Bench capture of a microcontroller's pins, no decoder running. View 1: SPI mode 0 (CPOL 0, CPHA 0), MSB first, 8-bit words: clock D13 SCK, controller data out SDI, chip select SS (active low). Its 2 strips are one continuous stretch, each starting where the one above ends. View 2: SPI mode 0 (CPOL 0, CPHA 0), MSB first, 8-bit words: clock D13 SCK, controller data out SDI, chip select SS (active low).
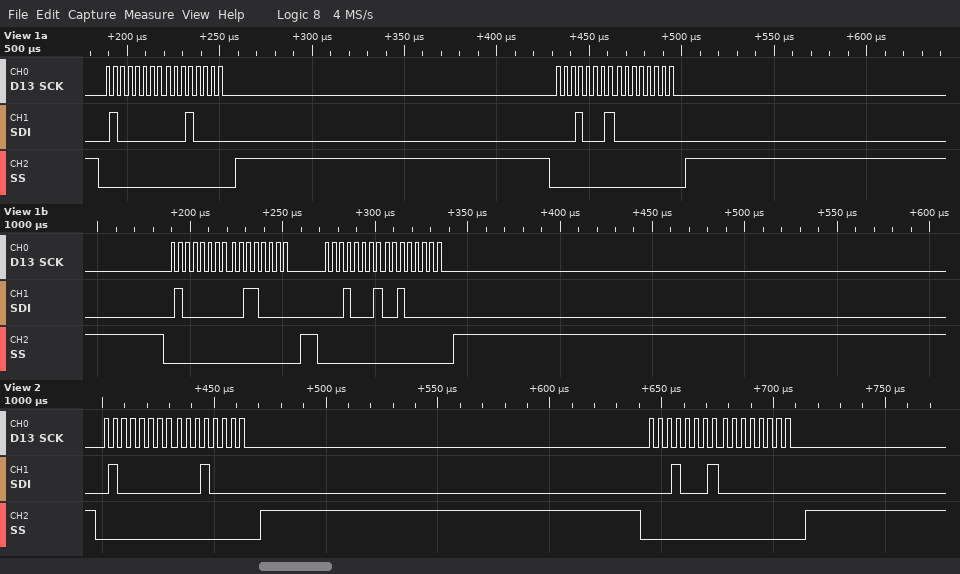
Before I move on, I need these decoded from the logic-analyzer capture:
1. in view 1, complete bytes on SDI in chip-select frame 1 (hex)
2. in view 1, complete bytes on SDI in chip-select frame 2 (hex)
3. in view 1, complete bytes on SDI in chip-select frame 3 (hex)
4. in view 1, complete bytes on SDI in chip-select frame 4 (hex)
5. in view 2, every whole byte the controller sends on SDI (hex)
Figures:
40 10
11 00
40 30
11 20
40 10 11 00
